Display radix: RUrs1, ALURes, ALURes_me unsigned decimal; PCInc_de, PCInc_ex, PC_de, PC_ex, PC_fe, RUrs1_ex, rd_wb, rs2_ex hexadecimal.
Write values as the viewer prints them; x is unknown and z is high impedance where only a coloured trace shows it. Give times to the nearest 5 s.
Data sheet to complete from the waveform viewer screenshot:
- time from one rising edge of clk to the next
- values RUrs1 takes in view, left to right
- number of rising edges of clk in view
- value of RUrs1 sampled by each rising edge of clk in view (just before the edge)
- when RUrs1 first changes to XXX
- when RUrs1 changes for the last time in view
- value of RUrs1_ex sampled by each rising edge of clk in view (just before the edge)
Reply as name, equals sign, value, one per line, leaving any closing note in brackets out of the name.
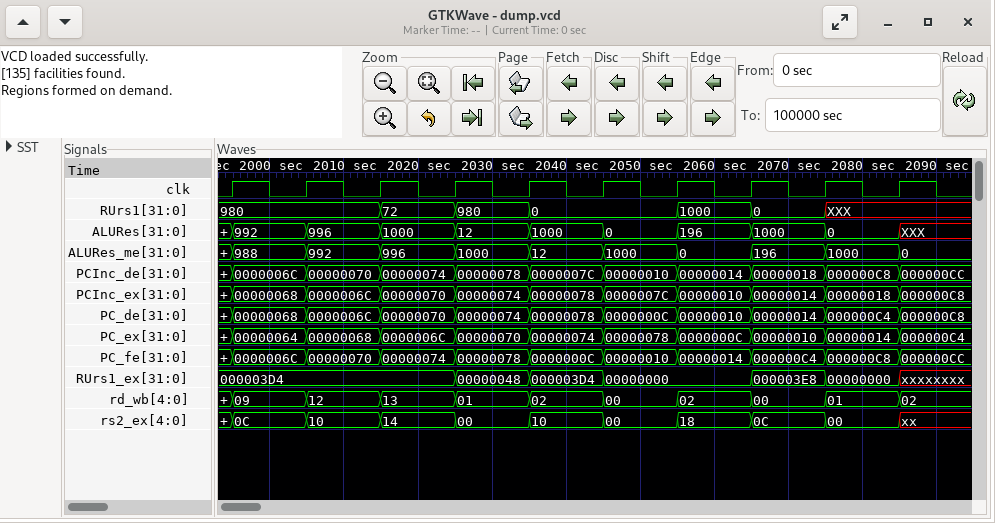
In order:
time from one rising edge of clk to the next = 10 s
values RUrs1 takes in view, left to right = 980, 72, 980, 0, 1000, 0, XXX
number of rising edges of clk in view = 10
value of RUrs1 sampled by each rising edge of clk in view = 980, 980, 980, 72, 980, 0, 0, 1000, 0, XXX
when RUrs1 first changes to XXX = 2075 s
when RUrs1 changes for the last time in view = 2075 s
value of RUrs1_ex sampled by each rising edge of clk in view = 000003D4, 000003D4, 000003D4, 000003D4, 00000048, 000003D4, 00000000, 00000000, 000003E8, 00000000
